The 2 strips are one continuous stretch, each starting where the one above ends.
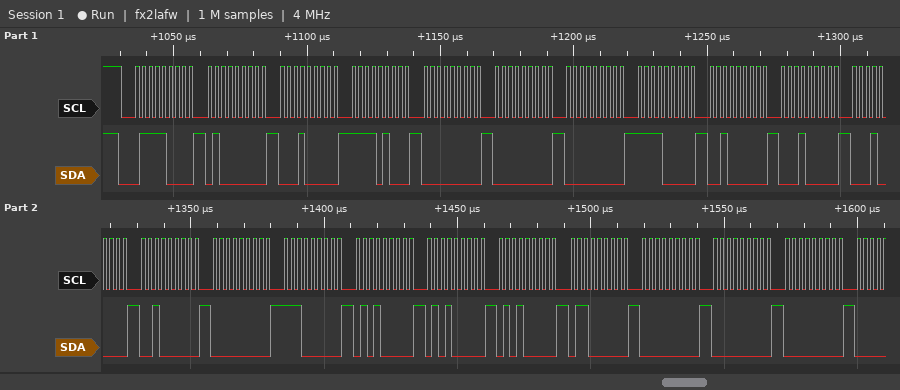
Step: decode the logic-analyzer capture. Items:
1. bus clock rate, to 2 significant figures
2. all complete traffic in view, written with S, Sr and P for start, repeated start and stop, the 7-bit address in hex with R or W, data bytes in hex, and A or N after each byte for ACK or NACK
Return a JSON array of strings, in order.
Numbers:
["400 kHz", "S 3CW A 40 A 10 A F4 A 00 A 00 A 00 A F0 A 20 A 10 A 10 A 20 A 00 A E0 A 50 A 50 A 50 A 60 A 00 A 00 A 00 A"]
